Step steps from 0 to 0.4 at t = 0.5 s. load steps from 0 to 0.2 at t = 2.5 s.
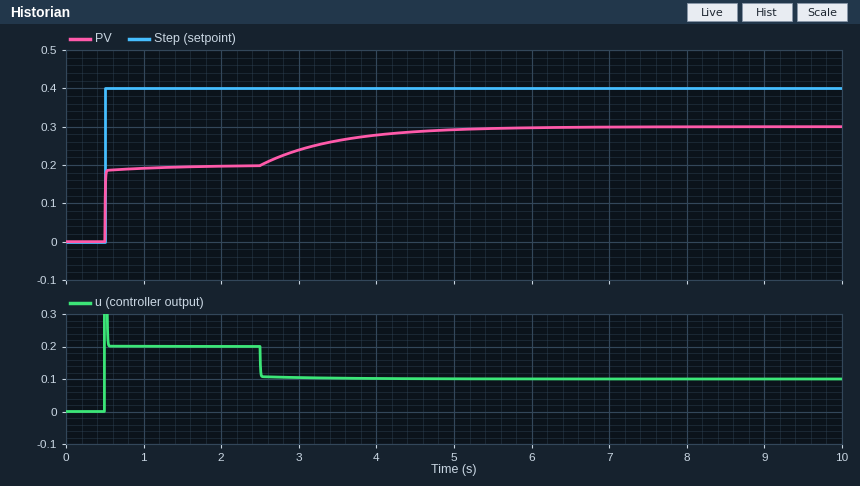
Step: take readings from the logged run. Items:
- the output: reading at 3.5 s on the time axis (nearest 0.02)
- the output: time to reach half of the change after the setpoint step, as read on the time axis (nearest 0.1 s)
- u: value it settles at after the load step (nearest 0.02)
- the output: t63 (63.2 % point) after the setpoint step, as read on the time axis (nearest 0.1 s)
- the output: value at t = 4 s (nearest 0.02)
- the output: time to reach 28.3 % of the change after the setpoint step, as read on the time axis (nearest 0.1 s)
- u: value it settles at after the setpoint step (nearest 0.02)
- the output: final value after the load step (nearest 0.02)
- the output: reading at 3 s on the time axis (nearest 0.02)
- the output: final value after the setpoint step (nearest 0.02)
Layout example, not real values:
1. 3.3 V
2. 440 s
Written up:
1. 0.26
2. 0.5 s
3. 0.10
4. 0.5 s
5. 0.28
6. 0.5 s
7. 0.20
8. 0.30
9. 0.24
10. 0.20
